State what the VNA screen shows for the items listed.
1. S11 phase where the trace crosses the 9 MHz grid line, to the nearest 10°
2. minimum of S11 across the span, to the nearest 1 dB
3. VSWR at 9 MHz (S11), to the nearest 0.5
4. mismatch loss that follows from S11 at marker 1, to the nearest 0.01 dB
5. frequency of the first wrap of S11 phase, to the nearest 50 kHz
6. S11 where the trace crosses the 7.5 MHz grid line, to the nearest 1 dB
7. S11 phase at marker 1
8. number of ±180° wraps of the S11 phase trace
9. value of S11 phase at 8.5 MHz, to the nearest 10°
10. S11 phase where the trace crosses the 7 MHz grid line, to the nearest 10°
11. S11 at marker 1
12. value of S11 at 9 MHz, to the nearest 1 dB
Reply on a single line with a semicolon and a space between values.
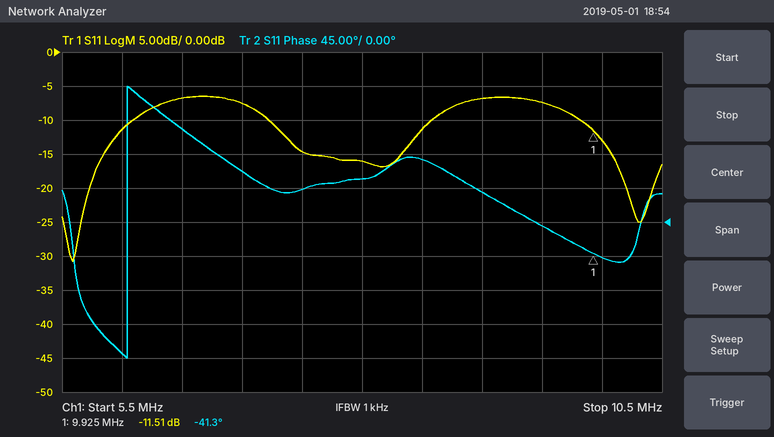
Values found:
40°; -31 dB; 2.5; 0.32 dB; 6.05 MHz; -15 dB; -41.3°; 1; 80°; 70°; -11.51 dB; -7 dB
